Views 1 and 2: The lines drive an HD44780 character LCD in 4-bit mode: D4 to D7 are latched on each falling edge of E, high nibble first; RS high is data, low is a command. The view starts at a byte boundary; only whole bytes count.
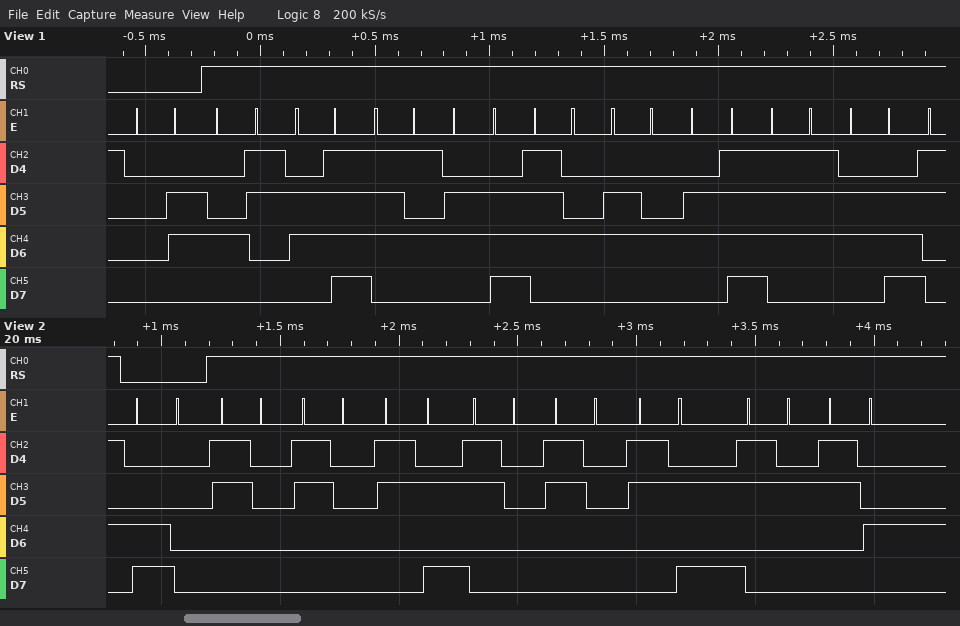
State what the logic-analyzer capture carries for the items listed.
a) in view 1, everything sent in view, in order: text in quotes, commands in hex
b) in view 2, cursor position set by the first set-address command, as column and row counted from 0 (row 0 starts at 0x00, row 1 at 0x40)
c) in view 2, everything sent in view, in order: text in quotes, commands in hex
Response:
0x06 "Countdown"
column 0, row 1
0xC0 "00:00:24"
